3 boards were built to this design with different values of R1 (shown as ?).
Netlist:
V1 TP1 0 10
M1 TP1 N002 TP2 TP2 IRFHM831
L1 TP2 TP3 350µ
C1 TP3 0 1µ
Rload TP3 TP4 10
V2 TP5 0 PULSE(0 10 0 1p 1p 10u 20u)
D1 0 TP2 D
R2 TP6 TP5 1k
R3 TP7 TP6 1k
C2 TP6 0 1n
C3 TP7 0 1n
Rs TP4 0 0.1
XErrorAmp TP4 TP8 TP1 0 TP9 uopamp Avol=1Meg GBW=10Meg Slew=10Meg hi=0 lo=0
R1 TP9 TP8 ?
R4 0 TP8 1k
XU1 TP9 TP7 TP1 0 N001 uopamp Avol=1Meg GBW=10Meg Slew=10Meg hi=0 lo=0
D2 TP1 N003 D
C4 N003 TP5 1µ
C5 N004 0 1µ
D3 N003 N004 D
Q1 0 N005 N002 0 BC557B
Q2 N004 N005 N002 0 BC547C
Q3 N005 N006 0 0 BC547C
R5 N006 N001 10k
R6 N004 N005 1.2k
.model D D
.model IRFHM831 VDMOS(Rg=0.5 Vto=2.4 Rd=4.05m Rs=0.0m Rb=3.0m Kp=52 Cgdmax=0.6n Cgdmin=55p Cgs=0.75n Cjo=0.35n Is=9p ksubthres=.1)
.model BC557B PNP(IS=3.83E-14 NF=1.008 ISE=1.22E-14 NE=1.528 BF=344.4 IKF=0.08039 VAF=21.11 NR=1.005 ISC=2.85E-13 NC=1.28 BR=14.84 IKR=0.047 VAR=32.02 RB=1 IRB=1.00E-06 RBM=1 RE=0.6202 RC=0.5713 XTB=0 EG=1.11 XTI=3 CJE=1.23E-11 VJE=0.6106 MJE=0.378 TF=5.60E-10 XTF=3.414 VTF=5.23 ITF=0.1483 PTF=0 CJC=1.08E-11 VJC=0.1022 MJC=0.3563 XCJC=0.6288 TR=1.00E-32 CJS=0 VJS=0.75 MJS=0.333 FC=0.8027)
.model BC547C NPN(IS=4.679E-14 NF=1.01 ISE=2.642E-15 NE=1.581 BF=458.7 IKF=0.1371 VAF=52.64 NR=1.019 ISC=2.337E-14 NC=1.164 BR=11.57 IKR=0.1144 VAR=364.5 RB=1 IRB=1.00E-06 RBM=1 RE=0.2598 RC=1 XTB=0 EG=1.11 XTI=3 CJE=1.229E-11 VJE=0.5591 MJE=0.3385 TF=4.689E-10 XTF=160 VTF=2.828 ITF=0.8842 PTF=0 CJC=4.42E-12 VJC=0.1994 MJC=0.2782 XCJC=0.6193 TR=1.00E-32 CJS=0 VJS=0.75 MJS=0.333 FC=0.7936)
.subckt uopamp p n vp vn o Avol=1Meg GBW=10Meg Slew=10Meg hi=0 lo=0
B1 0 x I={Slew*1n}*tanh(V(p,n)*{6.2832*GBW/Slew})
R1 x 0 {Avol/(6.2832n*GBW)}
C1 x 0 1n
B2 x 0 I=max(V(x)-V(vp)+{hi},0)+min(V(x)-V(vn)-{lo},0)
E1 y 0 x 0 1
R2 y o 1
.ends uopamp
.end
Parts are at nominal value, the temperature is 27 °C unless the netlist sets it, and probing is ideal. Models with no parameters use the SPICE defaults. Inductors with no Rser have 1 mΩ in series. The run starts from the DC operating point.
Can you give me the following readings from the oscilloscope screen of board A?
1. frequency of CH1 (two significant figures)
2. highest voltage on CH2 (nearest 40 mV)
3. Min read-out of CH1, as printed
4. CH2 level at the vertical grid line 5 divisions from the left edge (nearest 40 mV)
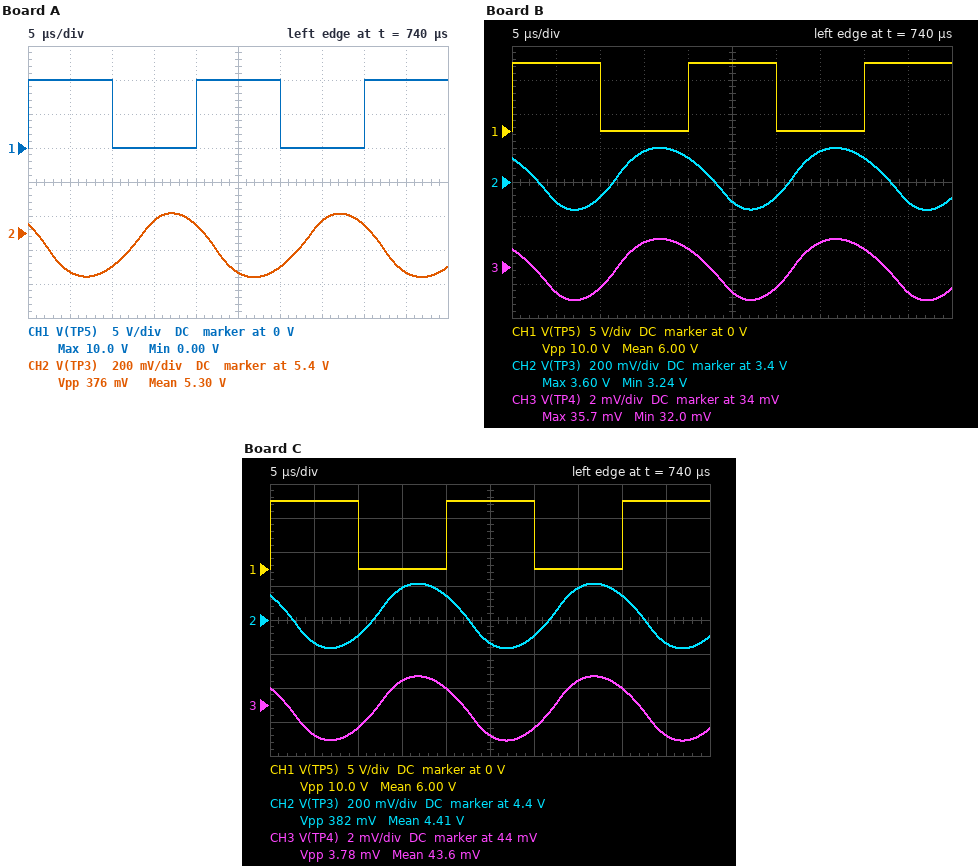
50 kHz
5.52 V
0.00 V
5.16 V
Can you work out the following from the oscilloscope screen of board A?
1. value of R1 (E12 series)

56 kΩ
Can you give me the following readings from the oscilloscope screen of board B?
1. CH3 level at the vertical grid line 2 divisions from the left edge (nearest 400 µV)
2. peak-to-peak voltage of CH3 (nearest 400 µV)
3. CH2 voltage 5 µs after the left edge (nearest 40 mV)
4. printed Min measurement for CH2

32.8 mV
3.6 mV
3.28 V
3.24 V
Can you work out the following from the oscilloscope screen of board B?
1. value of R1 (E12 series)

180 kΩ
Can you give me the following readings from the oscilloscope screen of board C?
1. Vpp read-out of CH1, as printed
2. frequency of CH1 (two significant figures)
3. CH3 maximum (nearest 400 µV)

10.0 V
50 kHz
45.6 mV
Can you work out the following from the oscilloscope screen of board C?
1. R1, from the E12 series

100 kΩ
